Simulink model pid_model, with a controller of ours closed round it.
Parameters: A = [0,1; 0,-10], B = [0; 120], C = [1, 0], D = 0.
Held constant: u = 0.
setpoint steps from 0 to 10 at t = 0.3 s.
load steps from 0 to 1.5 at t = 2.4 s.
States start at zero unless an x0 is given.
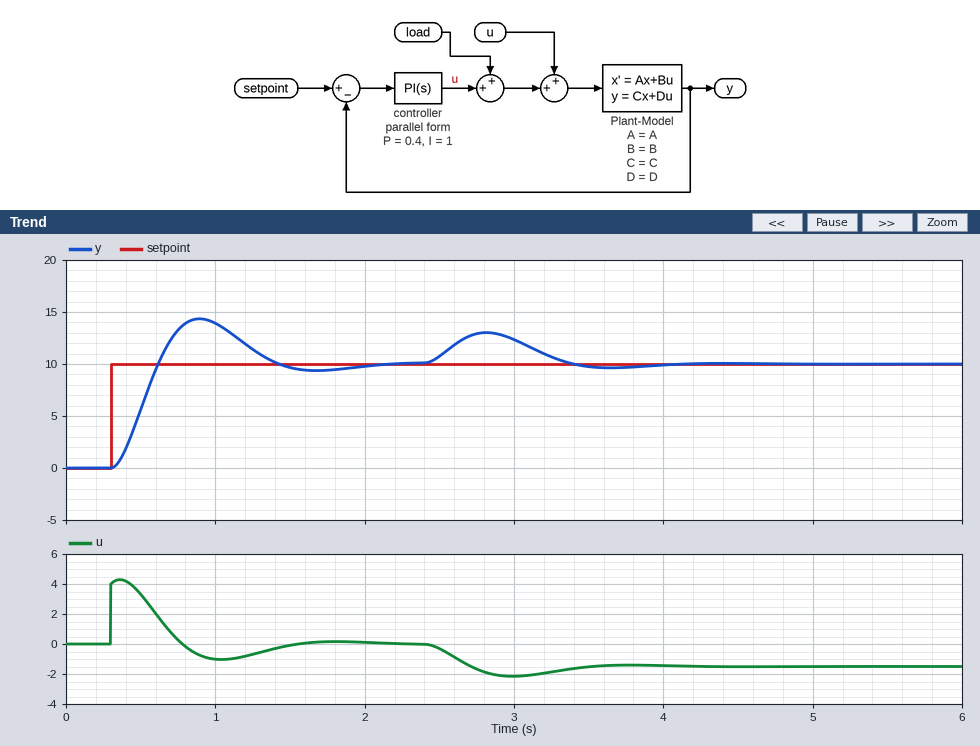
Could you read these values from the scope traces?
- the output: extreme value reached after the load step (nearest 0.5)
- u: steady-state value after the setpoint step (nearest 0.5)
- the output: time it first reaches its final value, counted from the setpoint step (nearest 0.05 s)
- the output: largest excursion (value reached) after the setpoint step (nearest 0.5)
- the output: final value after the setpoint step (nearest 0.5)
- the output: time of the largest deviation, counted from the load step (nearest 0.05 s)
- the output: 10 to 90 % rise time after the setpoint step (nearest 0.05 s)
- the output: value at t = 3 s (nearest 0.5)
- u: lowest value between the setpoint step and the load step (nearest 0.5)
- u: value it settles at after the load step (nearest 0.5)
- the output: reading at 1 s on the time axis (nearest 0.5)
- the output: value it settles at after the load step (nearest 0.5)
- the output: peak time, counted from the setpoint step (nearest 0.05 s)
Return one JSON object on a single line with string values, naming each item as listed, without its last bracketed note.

{"the output: extreme value reached after the load step": "13.0", "u: steady-state value after the setpoint step": "0.0", "the output: time it first reaches its final value, counted from the setpoint step": "0.30 s", "the output: largest excursion (value reached) after the setpoint step": "14.5", "the output: final value after the setpoint step": "10.0", "the output: time of the largest deviation, counted from the load step": "0.40 s", "the output: 10 to 90 % rise time after the setpoint step": "0.20 s", "the output: value at t = 3 s": "12.5", "u: lowest value between the setpoint step and the load step": "-1.0", "u: value it settles at after the load step": "-1.5", "the output: reading at 1 s on the time axis": "14.0", "the output: value it settles at after the load step": "10.0", "the output: peak time, counted from the setpoint step": "0.60 s"}
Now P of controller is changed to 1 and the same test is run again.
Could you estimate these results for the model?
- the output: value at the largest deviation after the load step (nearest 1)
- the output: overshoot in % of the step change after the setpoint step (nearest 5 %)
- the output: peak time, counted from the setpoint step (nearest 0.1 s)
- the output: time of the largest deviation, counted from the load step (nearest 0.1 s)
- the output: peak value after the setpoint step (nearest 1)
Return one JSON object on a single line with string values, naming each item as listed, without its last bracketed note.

{"the output: value at the largest deviation after the load step": "12", "the output: overshoot in % of the step change after the setpoint step": "30 %", "the output: peak time, counted from the setpoint step": "0.3 s", "the output: time of the largest deviation, counted from the load step": "0.3 s", "the output: peak value after the setpoint step": "13"}
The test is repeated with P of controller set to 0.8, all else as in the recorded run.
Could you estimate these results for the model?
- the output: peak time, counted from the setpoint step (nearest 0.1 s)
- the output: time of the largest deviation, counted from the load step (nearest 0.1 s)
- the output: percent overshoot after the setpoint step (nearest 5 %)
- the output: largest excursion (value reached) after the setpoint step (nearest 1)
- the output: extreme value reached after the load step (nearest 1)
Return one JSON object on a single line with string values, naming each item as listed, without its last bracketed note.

{"the output: peak time, counted from the setpoint step": "0.4 s", "the output: time of the largest deviation, counted from the load step": "0.3 s", "the output: percent overshoot after the setpoint step": "30 %", "the output: largest excursion (value reached) after the setpoint step": "13", "the output: extreme value reached after the load step": "12"}
